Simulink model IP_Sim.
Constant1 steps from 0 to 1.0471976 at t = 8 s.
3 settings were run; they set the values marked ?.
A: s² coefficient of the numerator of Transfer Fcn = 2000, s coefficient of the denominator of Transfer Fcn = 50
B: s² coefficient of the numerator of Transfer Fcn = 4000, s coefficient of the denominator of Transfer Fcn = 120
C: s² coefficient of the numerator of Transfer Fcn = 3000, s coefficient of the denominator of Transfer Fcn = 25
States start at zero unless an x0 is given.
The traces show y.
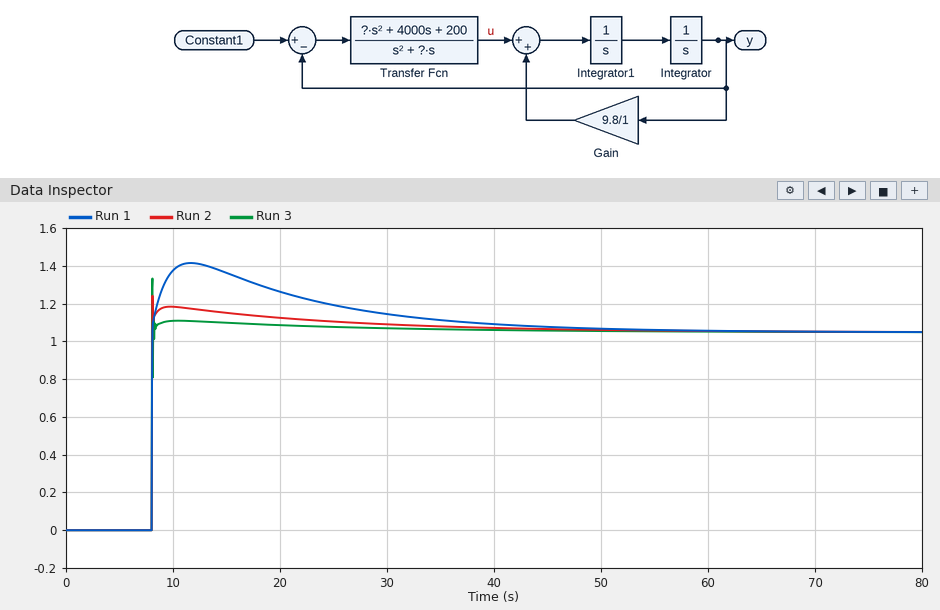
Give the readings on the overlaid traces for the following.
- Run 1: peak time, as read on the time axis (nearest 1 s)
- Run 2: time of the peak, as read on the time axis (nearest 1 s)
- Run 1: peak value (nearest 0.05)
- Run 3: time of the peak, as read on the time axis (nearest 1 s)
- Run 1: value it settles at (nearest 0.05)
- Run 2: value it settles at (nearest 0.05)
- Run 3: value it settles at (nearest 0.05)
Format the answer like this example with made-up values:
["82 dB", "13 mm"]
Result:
["12 s", "8 s", "1.40", "8 s", "1.05", "1.05", "1.05"]
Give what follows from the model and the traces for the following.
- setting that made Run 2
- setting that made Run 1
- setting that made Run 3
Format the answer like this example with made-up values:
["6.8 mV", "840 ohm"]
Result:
["A", "B", "C"]
